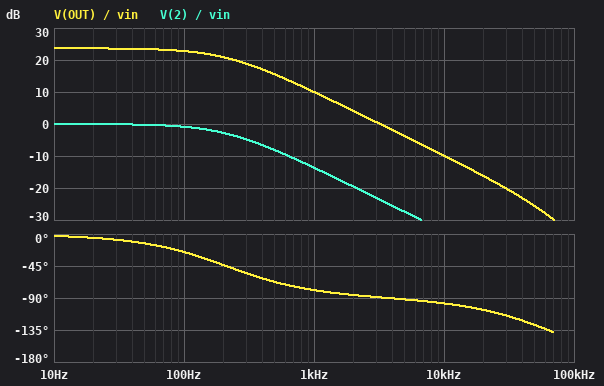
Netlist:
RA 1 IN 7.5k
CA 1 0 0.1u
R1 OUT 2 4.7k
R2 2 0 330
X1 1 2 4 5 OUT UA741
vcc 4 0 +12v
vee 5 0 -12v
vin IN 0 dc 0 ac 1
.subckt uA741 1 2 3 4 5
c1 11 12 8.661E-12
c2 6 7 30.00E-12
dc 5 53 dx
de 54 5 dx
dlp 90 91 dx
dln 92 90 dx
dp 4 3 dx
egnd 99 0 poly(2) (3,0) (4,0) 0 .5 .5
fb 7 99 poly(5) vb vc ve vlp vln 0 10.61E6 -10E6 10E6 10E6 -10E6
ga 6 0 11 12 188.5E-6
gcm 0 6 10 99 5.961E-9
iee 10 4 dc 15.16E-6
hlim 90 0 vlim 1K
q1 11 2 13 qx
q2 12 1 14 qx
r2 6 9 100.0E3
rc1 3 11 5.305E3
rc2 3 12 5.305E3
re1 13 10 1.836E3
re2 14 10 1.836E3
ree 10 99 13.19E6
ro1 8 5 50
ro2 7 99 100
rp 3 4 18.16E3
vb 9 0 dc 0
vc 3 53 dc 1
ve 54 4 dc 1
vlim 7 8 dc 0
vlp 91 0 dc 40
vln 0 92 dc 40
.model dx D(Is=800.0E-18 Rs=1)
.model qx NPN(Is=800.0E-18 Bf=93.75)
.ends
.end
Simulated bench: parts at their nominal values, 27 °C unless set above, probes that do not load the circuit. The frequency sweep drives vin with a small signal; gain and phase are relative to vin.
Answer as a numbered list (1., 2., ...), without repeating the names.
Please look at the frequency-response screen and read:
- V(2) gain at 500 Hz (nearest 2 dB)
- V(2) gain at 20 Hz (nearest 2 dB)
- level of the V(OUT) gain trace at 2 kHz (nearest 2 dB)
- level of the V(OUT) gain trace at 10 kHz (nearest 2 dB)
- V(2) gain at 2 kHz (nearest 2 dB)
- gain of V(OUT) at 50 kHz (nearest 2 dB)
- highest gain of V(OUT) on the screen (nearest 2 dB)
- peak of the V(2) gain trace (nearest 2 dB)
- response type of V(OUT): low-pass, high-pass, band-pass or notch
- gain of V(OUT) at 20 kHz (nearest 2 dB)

1. -8 dB
2. 0 dB
3. 4 dB
4. -10 dB
5. -20 dB
6. -26 dB
7. 24 dB
8. 0 dB
9. low-pass
10. -16 dB
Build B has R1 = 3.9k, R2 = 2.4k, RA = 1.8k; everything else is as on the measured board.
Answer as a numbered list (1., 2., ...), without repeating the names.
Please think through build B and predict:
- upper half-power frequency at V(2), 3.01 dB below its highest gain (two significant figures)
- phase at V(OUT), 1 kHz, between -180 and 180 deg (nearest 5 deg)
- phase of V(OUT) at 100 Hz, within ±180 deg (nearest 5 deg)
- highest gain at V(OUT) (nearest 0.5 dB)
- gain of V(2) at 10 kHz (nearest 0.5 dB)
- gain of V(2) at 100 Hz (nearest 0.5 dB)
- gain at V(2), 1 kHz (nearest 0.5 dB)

1. 880 Hz
2. -50 deg
3. -5 deg
4. 8.5 dB
5. -21.0 dB
6. 0 dB
7. -3.5 dB
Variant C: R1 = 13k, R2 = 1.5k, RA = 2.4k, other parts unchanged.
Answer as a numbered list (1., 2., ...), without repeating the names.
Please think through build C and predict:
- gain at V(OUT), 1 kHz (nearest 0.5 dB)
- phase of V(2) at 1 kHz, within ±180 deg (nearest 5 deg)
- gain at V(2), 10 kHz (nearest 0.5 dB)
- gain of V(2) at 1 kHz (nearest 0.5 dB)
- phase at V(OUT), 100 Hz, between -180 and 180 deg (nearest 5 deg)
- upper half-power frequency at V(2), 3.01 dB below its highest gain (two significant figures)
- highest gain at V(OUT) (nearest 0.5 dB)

1. 14.5 dB
2. -55 deg
3. -23.5 dB
4. -5.0 dB
5. -10 deg
6. 660 Hz
7. 19.5 dB
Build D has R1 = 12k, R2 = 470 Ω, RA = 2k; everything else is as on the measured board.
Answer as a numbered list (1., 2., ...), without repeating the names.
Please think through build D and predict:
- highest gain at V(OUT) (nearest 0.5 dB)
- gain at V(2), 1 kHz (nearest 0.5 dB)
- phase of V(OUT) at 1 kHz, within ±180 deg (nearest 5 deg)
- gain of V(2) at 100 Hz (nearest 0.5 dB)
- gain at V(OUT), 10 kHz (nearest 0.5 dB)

1. 28.5 dB
2. -4.0 dB
3. -55 deg
4. 0 dB
5. 6.0 dB
